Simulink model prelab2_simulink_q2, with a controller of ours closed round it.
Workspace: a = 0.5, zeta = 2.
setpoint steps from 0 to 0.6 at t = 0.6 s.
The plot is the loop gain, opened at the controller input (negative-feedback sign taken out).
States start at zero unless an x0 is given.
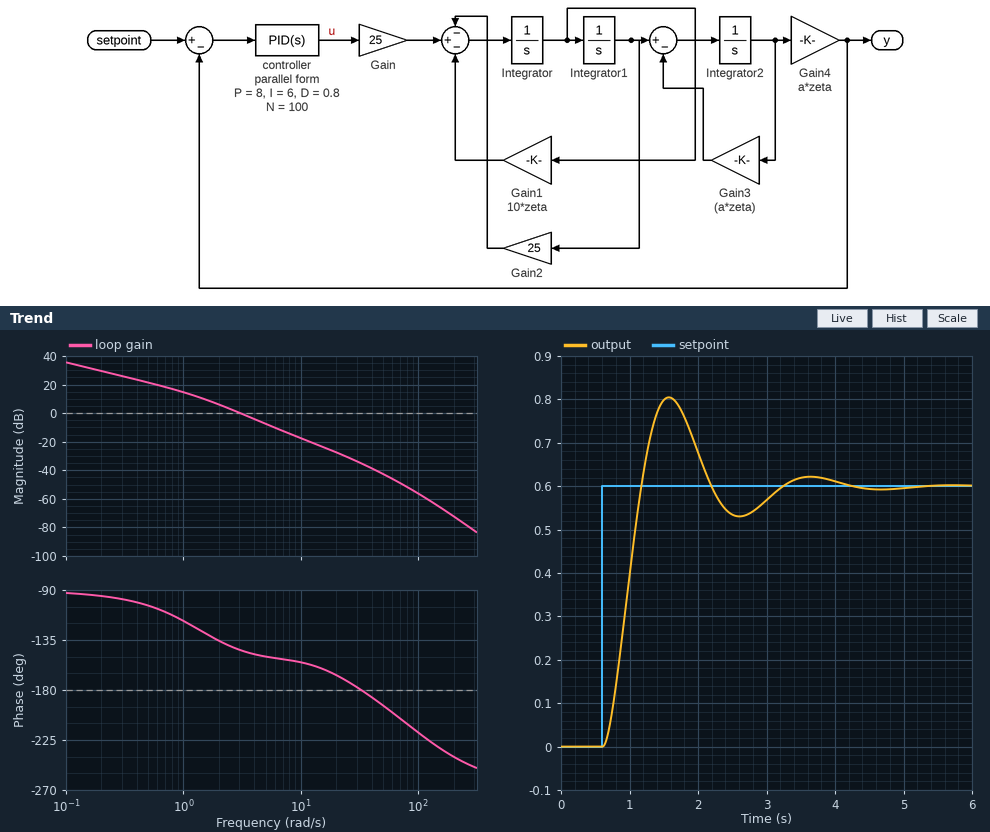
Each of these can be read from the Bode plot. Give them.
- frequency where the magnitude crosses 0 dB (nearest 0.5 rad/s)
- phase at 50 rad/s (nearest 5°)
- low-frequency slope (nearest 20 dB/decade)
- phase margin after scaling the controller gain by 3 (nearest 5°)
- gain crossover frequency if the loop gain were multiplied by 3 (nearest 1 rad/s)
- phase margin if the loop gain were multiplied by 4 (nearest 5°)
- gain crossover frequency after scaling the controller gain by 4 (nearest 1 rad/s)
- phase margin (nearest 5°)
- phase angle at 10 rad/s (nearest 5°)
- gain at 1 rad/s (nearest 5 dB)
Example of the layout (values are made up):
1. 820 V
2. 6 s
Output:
1. 3.0 rad/s
2. -195°
3. -20 dB/decade
4. 30°
5. 6 rad/s
6. 30°
7. 7 rad/s
8. 35°
9. -155°
10. 15 dB
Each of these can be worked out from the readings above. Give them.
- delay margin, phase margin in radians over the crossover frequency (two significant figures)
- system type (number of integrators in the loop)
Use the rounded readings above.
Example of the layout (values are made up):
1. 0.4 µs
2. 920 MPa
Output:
1. 0.20 s
2. 1
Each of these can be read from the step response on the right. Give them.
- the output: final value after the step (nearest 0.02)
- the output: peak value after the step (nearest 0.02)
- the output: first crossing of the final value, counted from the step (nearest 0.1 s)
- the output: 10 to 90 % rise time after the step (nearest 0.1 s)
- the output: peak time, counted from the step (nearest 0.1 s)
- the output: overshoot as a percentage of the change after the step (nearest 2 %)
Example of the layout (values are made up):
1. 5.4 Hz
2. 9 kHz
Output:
1. 0.60
2. 0.80
3. 0.6 s
4. 0.4 s
5. 1.0 s
6. 34 %
